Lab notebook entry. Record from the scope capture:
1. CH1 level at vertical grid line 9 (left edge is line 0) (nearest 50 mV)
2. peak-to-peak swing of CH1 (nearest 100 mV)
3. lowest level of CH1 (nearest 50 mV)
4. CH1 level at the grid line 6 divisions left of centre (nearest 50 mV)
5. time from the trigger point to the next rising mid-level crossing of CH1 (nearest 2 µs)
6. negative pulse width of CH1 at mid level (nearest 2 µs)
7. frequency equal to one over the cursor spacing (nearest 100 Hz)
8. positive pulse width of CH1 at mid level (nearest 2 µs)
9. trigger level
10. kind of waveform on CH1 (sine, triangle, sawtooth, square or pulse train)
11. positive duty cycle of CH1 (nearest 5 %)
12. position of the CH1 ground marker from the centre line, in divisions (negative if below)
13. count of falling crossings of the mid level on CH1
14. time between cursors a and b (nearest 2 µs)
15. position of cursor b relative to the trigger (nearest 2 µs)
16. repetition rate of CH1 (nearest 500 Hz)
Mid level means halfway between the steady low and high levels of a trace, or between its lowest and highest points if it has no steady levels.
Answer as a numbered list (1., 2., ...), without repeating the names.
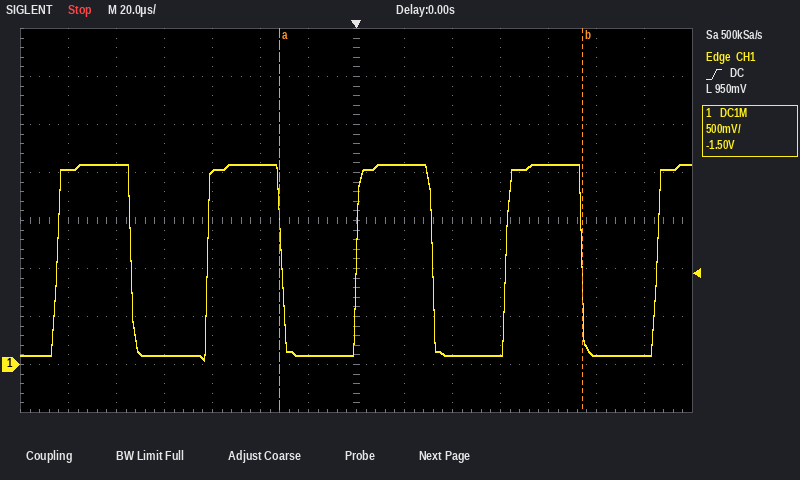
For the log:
1. 100 mV
2. 2.00 V
3. 50 mV
4. 2.05 V
5. 62 µs
6. 32 µs
7. 7.9 kHz
8. 32 µs
9. 950 mV
10. square
11. 50 %
12. -3.0 div
13. 4
14. 126 µs
15. +94 µs
16. 16.0 kHz
